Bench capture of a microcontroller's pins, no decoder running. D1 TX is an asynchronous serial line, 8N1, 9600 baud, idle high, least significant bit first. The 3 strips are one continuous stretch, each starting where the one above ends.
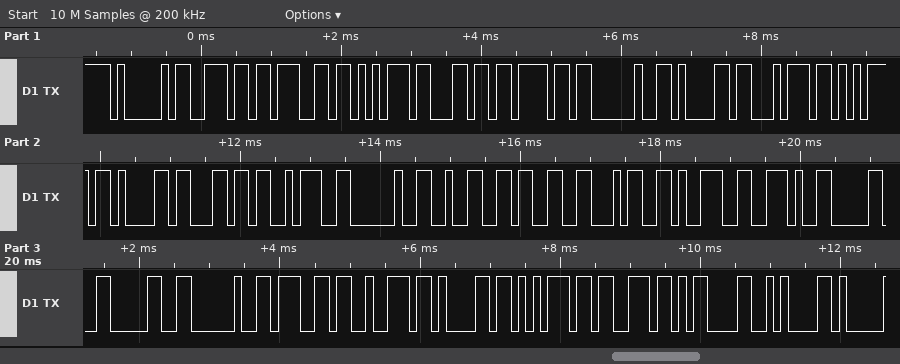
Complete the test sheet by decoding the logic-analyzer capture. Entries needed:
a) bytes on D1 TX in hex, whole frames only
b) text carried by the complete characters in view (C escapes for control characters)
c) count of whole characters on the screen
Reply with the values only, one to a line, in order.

0x41 0x6E 0x67 0x75 0x6C 0x6F 0x20 0x61 0x74 0x75 0x61 0x6C 0x3A 0x20 0x32 0x33 0x34 0x39 0x2E 0x30 0x30 0x20 0x67 0x72 0x61 0x75 0x73 0x0D 0x0A
"Angulo atual: 2349.00 graus\r\n"
29
